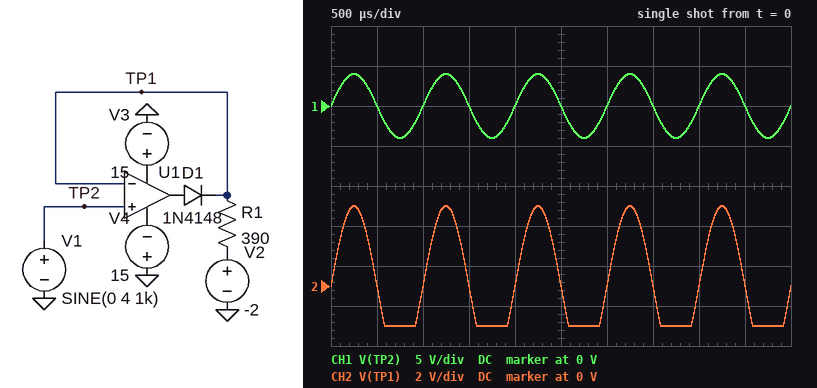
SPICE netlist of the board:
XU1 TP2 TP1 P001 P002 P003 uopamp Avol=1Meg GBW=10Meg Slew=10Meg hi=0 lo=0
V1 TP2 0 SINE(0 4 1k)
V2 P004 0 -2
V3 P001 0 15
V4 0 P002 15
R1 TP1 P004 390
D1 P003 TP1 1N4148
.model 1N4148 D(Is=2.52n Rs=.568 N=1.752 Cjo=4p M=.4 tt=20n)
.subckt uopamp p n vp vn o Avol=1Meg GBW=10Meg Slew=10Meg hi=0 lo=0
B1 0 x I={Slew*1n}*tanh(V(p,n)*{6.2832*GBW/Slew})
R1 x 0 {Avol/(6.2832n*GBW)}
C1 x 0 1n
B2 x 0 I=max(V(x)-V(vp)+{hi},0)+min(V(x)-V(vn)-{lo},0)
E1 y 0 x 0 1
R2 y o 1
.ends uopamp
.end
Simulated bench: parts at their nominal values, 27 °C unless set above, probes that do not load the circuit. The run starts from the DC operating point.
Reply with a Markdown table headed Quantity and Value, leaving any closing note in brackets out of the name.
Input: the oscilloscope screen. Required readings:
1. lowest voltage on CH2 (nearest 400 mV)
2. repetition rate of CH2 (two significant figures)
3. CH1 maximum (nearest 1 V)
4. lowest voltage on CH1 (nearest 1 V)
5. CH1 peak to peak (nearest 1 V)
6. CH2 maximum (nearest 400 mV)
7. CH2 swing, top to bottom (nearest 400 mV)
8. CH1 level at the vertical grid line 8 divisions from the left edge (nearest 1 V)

| Quantity | Value |
|---|---|
| lowest voltage on CH2 | -2.0 V |
| repetition rate of CH2 | 1.0 kHz |
| CH1 maximum | 4 V |
| lowest voltage on CH1 | -4 V |
| CH1 peak to peak | 8 V |
| CH2 maximum | 4.0 V |
| CH2 swing, top to bottom | 6.0 V |
| CH1 level at the vertical grid line 8 divisions from the left edge | 0 V |
